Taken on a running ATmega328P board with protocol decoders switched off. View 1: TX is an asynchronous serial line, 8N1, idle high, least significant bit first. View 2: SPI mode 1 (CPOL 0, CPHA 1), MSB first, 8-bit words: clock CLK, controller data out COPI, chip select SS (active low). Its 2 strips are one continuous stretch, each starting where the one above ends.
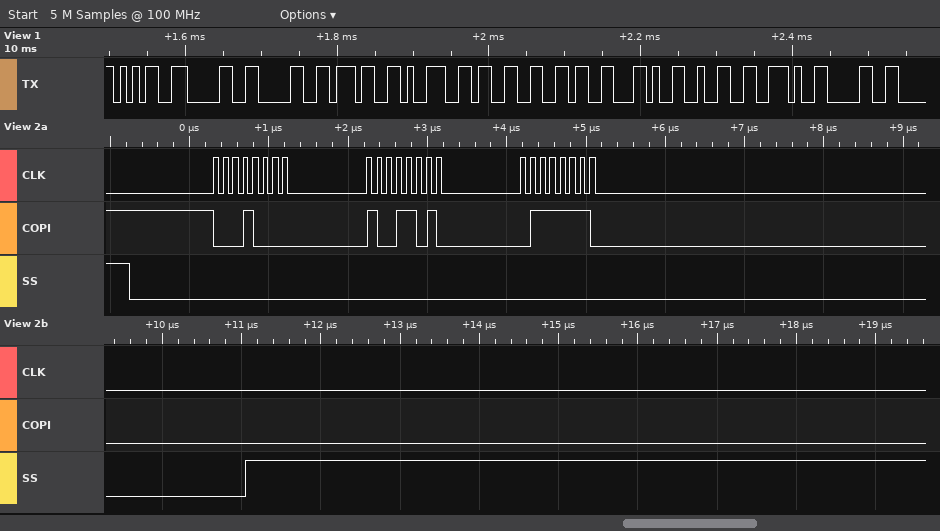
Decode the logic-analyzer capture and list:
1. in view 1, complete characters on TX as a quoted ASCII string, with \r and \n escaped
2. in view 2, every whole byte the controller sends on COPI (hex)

"5007936,2.0"
0x10 0x9A 0x7E
